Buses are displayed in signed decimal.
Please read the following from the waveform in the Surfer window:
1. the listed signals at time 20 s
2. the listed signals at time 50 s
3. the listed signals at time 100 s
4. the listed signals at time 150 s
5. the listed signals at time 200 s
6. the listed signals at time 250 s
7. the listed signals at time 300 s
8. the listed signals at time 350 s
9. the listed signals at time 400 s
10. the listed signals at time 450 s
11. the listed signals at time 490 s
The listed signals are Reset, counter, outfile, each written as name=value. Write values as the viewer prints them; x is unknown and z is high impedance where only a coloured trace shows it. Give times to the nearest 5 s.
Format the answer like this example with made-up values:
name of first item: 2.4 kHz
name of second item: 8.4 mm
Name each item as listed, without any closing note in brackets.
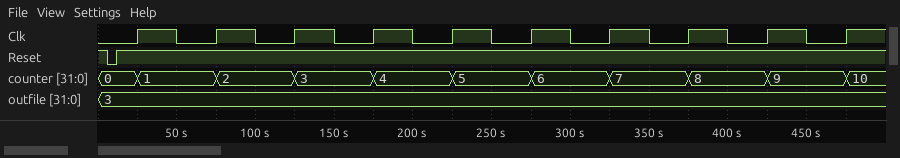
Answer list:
the listed signals at time 20 s: Reset=1, counter=0, outfile=3
the listed signals at time 50 s: Reset=1, counter=1, outfile=3
the listed signals at time 100 s: Reset=1, counter=2, outfile=3
the listed signals at time 150 s: Reset=1, counter=3, outfile=3
the listed signals at time 200 s: Reset=1, counter=4, outfile=3
the listed signals at time 250 s: Reset=1, counter=5, outfile=3
the listed signals at time 300 s: Reset=1, counter=6, outfile=3
the listed signals at time 350 s: Reset=1, counter=7, outfile=3
the listed signals at time 400 s: Reset=1, counter=8, outfile=3
the listed signals at time 450 s: Reset=1, counter=9, outfile=3
the listed signals at time 490 s: Reset=1, counter=10, outfile=3
